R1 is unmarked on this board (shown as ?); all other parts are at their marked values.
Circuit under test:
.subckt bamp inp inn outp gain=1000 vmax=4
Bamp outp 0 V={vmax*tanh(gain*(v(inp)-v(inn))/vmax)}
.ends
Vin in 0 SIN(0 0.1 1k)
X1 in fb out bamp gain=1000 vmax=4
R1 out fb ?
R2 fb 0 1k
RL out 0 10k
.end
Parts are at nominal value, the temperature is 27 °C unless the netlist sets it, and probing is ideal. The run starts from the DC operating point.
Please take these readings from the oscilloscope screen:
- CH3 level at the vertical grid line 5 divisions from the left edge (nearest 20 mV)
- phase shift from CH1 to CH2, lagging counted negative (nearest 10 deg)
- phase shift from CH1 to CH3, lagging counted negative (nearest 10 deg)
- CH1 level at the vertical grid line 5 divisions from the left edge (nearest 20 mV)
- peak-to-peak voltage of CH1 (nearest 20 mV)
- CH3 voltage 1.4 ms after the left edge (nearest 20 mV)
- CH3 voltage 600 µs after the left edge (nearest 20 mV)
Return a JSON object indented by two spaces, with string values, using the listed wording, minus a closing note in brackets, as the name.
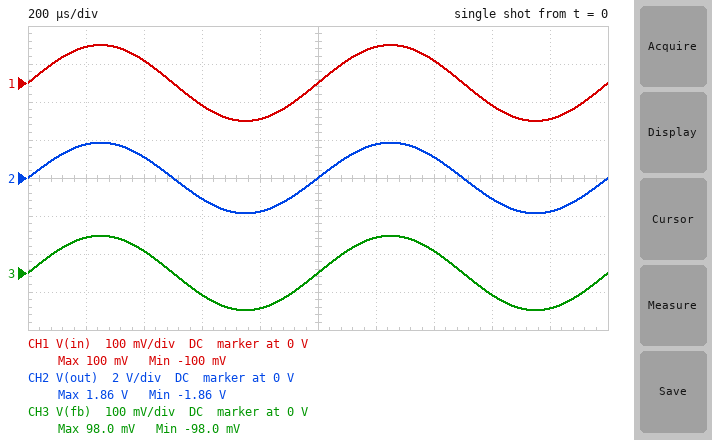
{
  "CH3 level at the vertical grid line 5 divisions from the left edge": "0 V",
  "phase shift from CH1 to CH2, lagging counted negative": "0 deg",
  "phase shift from CH1 to CH3, lagging counted negative": "0 deg",
  "CH1 level at the vertical grid line 5 divisions from the left edge": "0 V",
  "peak-to-peak voltage of CH1": "200 mV",
  "CH3 voltage 1.4 ms after the left edge": "60 mV",
  "CH3 voltage 600 µs after the left edge": "-60 mV"
}
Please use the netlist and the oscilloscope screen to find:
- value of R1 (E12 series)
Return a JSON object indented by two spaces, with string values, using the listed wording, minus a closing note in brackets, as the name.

{
  "value of R1": "18 kΩ"
}
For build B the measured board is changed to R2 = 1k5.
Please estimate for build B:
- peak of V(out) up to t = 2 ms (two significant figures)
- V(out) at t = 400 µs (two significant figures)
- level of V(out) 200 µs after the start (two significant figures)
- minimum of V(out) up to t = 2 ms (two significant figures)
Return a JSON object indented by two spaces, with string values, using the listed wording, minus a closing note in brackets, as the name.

{
  "peak of V(out) up to t = 2 ms": "1.3 V",
  "V(out) at t = 400 µs": "750 mV",
  "level of V(out) 200 µs after the start": "1.2 V",
  "minimum of V(out) up to t = 2 ms": "-1.3 V"
}
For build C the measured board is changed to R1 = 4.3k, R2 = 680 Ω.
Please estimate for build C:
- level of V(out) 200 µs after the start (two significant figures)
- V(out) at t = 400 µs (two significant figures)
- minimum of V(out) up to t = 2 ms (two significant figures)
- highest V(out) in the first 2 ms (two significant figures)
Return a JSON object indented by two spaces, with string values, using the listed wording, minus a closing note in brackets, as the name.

{
  "level of V(out) 200 µs after the start": "690 mV",
  "V(out) at t = 400 µs": "430 mV",
  "minimum of V(out) up to t = 2 ms": "-730 mV",
  "highest V(out) in the first 2 ms": "730 mV"
}
